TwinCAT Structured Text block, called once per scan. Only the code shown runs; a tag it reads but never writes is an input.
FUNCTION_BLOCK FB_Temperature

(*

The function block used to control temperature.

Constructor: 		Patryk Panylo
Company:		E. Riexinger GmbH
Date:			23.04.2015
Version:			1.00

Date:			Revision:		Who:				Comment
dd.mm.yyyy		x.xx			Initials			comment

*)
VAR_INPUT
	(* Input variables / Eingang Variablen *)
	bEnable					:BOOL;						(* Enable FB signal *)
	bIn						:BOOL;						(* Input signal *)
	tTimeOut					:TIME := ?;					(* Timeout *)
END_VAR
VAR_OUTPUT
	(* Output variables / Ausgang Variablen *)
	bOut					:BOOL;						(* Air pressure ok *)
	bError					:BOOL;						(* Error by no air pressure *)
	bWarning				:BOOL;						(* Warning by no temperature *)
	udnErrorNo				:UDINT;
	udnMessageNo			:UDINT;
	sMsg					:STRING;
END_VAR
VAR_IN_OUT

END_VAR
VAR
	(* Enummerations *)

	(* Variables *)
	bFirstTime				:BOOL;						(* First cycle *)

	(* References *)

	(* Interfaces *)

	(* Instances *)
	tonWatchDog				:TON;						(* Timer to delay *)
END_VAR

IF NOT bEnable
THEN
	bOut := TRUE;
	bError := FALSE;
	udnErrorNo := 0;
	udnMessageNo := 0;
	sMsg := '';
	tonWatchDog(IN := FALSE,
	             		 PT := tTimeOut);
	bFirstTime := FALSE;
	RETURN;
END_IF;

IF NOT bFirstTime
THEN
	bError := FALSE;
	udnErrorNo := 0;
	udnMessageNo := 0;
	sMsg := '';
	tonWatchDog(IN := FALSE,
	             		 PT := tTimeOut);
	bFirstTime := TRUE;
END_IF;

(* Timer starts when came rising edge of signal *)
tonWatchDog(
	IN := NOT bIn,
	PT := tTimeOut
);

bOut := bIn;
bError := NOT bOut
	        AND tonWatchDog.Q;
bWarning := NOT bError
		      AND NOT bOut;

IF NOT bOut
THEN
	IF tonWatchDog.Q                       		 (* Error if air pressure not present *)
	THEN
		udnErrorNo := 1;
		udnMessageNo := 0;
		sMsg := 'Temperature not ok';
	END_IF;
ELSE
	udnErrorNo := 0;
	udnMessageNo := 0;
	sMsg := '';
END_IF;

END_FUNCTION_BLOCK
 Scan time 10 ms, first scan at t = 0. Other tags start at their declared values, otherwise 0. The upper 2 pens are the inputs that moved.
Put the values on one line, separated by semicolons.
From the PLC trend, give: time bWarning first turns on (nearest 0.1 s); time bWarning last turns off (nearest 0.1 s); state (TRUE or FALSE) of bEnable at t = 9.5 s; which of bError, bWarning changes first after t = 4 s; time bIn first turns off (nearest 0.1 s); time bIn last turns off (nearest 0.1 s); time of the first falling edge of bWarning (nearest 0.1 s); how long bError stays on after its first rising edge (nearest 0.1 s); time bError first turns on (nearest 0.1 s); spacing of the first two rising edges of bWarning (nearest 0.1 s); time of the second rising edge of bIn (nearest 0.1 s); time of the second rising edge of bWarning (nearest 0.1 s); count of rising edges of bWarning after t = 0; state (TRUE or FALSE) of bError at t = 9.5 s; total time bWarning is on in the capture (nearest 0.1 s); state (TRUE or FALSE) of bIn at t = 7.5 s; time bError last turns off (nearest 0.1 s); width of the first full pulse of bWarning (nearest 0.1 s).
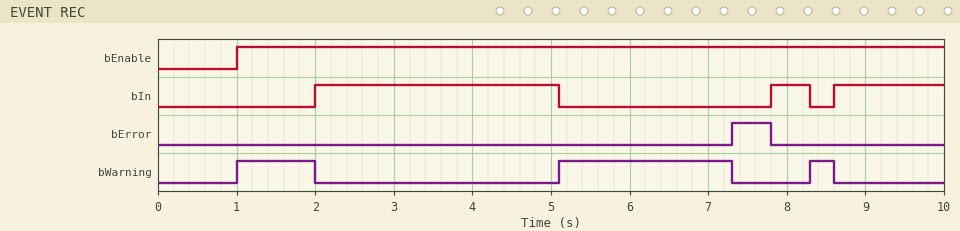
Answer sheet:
1.0 s; 8.6 s; TRUE; bWarning; 5.1 s; 8.3 s; 2.0 s; 0.5 s; 7.3 s; 4.1 s; 7.8 s; 5.1 s; 3; FALSE; 3.5 s; FALSE; 7.8 s; 1.0 s
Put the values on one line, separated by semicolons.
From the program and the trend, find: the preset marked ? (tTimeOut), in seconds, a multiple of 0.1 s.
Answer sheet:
2.2 s
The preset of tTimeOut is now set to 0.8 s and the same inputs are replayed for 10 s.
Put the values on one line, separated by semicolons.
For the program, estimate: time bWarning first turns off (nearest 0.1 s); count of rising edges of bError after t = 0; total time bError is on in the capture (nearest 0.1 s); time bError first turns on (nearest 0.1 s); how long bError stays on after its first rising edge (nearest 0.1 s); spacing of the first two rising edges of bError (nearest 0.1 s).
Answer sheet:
1.8 s; 2; 2.1 s; 1.8 s; 0.2 s; 4.1 s
